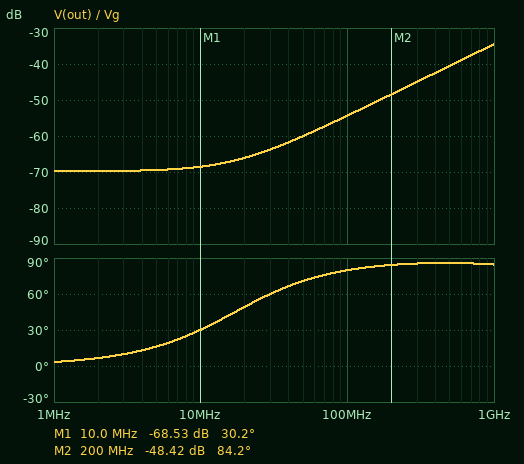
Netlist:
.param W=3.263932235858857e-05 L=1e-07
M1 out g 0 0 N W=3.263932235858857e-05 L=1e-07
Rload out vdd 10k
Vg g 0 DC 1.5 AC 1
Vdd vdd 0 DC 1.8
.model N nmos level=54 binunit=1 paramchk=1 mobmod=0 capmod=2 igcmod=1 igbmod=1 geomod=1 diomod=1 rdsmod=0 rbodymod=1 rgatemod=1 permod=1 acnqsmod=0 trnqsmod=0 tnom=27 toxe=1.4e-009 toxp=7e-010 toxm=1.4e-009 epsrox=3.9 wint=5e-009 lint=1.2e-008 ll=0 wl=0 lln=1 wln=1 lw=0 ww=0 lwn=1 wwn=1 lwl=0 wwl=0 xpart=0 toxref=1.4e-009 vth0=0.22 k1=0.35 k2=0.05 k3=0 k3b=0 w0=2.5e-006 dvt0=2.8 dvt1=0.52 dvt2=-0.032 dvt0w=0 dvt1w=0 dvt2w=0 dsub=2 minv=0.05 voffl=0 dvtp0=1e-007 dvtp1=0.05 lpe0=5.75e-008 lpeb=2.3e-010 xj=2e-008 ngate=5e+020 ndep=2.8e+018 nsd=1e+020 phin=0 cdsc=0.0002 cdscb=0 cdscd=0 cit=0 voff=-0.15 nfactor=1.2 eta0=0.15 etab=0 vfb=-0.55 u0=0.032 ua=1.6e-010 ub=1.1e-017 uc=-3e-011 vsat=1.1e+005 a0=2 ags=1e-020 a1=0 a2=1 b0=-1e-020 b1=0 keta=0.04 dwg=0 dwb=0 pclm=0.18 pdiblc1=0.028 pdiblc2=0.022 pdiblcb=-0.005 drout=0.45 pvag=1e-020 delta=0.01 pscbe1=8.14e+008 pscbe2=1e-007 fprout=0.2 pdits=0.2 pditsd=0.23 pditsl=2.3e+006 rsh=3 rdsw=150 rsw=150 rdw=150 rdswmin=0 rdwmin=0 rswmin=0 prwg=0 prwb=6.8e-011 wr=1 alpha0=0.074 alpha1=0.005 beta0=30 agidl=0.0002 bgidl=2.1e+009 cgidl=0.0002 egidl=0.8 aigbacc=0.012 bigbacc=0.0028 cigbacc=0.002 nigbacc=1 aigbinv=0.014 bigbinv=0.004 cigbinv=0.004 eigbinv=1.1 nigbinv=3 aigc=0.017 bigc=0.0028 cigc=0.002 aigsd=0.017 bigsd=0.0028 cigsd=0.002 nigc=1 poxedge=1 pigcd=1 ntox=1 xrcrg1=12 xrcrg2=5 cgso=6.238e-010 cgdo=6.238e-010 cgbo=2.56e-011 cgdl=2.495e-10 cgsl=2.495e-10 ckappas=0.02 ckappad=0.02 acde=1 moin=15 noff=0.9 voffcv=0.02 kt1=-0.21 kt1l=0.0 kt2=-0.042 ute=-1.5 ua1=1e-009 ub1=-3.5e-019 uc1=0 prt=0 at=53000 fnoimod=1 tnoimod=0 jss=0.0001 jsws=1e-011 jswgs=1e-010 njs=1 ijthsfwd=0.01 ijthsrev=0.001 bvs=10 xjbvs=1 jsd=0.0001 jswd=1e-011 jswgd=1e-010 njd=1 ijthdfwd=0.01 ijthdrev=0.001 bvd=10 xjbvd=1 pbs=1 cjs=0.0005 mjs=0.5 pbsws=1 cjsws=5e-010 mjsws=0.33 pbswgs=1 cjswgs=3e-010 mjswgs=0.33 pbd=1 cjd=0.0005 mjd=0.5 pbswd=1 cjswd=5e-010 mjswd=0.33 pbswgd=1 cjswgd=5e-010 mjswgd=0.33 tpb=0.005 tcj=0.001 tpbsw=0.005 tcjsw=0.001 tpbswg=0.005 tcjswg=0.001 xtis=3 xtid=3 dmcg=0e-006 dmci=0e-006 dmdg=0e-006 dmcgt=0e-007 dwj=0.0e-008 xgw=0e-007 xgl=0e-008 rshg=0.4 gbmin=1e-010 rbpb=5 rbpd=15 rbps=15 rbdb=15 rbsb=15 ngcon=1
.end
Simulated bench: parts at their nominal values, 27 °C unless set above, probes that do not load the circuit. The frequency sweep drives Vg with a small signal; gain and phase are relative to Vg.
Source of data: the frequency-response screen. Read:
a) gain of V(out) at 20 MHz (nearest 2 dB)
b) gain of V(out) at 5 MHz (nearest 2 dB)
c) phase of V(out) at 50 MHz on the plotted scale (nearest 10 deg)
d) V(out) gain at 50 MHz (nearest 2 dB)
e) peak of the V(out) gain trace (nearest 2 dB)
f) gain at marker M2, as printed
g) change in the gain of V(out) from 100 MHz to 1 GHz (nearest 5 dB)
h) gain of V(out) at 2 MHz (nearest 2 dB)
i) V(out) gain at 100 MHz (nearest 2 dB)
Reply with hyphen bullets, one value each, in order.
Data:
- -66 dB
- -70 dB
- 70 deg
- -60 dB
- -34 dB
- -48.42 dB
- 20 dB
- -70 dB
- -54 dB
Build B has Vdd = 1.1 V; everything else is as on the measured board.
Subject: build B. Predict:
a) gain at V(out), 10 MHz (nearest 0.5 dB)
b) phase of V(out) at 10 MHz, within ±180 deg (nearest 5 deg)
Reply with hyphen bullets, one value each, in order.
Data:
- -70.0 dB
- 35 deg
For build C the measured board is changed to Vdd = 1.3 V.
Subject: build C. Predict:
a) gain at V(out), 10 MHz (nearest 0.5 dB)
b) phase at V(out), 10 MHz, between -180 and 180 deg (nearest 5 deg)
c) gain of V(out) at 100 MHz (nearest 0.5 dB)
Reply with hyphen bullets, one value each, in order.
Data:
- -69.5 dB
- 35 deg
- -54.5 dB
